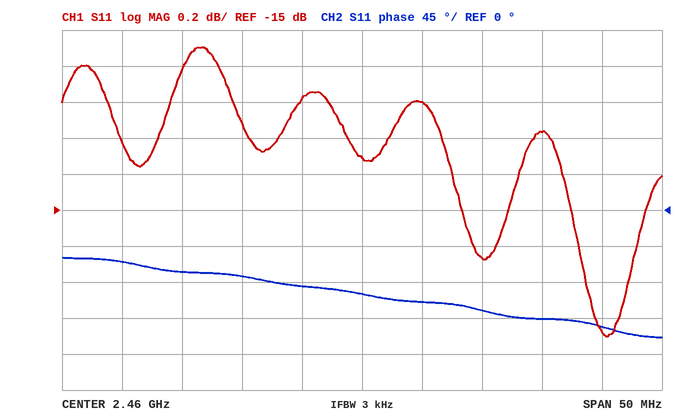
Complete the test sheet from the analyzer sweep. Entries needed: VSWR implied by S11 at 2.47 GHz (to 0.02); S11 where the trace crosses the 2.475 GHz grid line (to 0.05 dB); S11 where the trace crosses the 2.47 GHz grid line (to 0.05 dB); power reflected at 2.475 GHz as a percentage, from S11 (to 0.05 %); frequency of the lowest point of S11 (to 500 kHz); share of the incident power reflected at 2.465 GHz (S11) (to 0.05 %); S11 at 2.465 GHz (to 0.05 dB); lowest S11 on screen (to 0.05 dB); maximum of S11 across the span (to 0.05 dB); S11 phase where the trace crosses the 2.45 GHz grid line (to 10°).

1.42
-14.55 dB
-15.25 dB
3.50 %
2.4805 GHz
3.65 %
-14.40 dB
-15.70 dB
-14.10 dB
-80°
